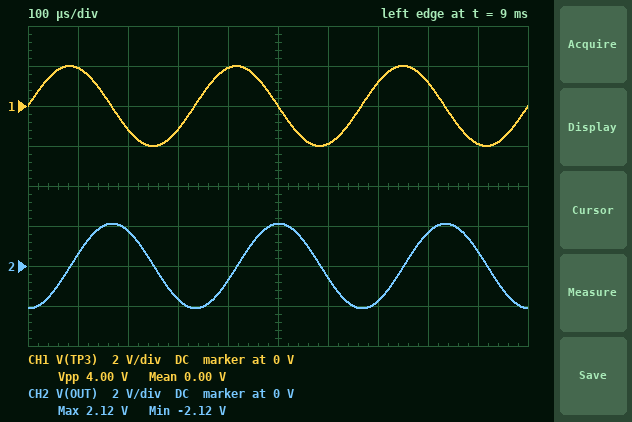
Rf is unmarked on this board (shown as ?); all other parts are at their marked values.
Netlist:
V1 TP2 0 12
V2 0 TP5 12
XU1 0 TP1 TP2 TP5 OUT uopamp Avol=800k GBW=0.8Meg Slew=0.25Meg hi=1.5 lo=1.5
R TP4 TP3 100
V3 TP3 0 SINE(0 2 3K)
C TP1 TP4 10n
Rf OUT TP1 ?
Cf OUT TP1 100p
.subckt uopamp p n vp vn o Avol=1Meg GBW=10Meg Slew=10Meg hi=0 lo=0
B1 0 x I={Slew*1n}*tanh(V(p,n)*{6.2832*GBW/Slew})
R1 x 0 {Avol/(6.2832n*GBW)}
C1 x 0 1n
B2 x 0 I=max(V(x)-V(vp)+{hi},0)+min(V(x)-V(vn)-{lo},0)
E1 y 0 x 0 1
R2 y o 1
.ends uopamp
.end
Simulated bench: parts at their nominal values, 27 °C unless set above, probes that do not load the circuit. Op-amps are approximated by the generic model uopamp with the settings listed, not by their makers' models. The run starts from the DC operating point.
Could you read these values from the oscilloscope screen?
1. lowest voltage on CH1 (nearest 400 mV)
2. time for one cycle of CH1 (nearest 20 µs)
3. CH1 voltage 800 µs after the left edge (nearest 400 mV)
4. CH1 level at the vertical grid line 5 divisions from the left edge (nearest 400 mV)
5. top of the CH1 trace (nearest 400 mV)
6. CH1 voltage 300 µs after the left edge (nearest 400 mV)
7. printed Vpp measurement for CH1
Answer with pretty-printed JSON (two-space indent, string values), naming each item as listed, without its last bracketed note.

{
  "lowest voltage on CH1": "-2.0 V",
  "time for one cycle of CH1": "340 µs",
  "CH1 voltage 800 µs after the left edge": "1.2 V",
  "CH1 level at the vertical grid line 5 divisions from the left edge": "0 V",
  "top of the CH1 trace": "2.0 V",
  "CH1 voltage 300 µs after the left edge": "-1.2 V",
  "printed Vpp measurement for CH1": "4.00 V"
}
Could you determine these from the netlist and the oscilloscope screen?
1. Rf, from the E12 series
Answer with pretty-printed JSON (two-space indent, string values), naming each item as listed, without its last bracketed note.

{
  "Rf, from the E12 series": "5.6 kΩ"
}
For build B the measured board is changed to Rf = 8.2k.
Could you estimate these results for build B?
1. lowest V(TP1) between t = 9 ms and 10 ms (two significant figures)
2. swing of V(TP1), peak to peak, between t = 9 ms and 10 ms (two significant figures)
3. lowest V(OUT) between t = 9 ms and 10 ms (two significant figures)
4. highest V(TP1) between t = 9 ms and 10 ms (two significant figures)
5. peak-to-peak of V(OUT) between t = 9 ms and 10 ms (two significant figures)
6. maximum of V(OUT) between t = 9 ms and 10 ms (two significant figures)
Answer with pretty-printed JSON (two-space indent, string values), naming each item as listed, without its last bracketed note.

{
  "lowest V(TP1) between t = 9 ms and 10 ms": "-12 mV",
  "swing of V(TP1), peak to peak, between t = 9 ms and 10 ms": "24 mV",
  "lowest V(OUT) between t = 9 ms and 10 ms": "-3.1 V",
  "highest V(TP1) between t = 9 ms and 10 ms": "12 mV",
  "peak-to-peak of V(OUT) between t = 9 ms and 10 ms": "6.2 V",
  "maximum of V(OUT) between t = 9 ms and 10 ms": "3.1 V"
}
